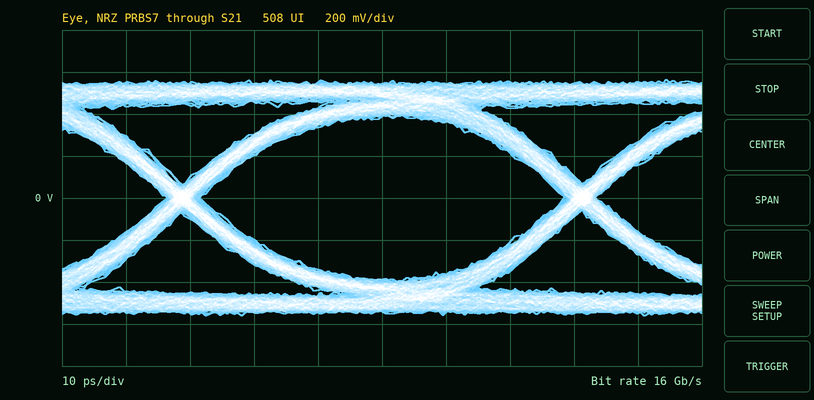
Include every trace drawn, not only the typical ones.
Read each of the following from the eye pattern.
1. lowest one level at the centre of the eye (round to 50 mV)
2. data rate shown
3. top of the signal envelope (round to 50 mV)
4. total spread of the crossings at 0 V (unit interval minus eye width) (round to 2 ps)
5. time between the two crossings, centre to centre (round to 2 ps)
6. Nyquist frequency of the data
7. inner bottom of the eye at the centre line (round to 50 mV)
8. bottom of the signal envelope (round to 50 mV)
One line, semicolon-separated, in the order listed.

400 mV; 16 Gb/s; 550 mV; 6 ps; 62 ps; 8 GHz; -400 mV; -550 mV
